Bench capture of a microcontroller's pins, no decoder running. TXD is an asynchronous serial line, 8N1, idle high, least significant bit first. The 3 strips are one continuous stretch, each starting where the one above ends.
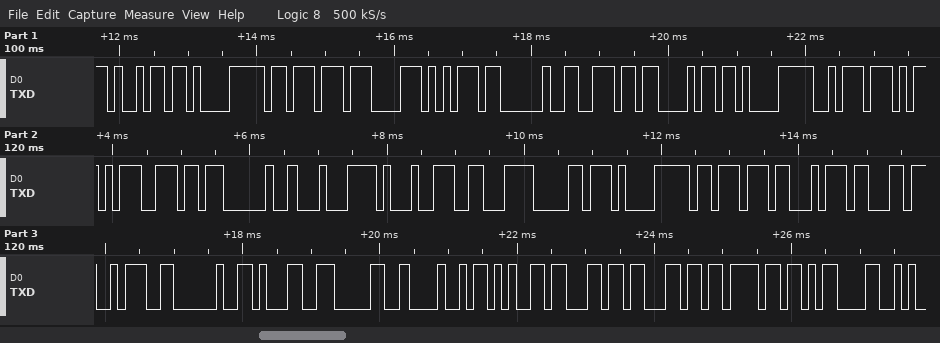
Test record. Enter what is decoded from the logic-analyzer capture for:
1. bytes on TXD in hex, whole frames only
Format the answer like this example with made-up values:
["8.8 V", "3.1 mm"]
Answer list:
["69 E1 BB 87 75 20 6E 68 E1 BA AD 6E 20 C4 91 C6 B0 E1 BB A3 63 3A 20 31 30 48 65 6C 6C 6F 0D"]
